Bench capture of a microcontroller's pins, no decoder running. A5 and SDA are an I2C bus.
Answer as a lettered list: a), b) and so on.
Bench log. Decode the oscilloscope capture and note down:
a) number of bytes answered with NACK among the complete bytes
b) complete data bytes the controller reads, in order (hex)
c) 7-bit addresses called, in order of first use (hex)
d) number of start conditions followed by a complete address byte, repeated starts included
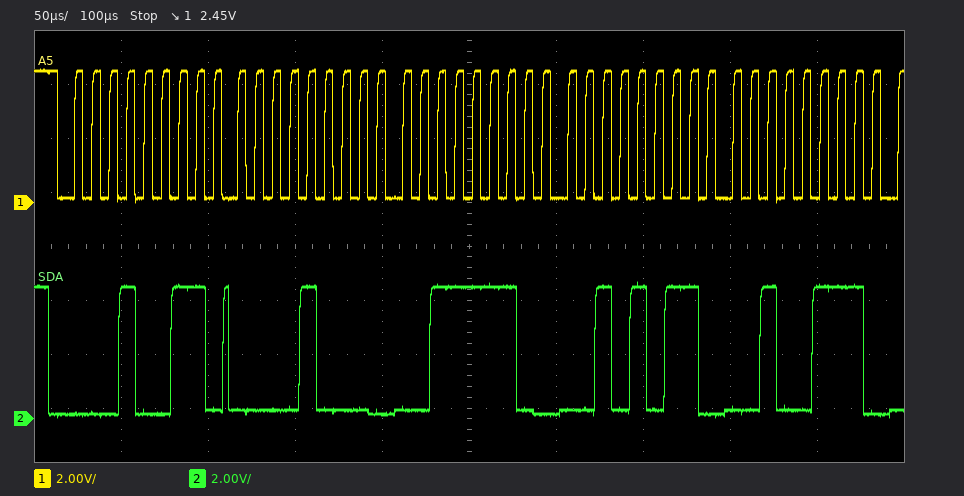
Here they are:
a) 0
b) 08 3E 2B 27
c) 0x09
d) 1
